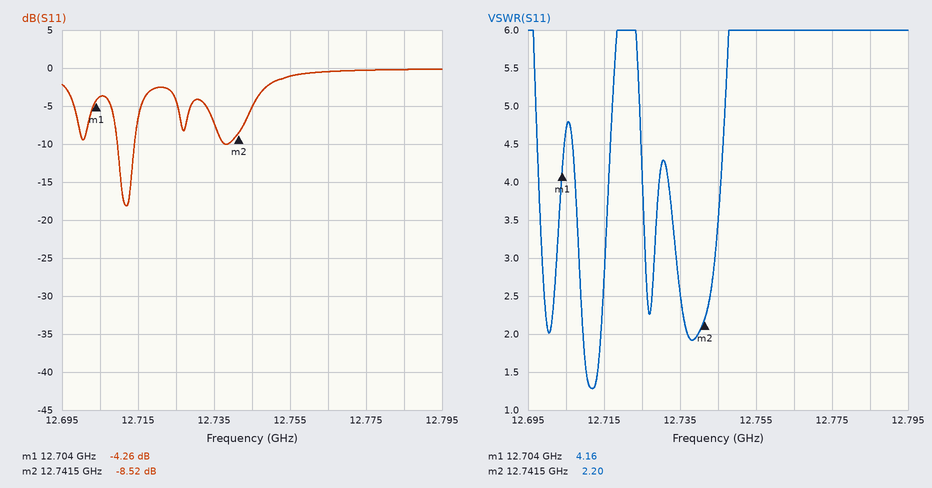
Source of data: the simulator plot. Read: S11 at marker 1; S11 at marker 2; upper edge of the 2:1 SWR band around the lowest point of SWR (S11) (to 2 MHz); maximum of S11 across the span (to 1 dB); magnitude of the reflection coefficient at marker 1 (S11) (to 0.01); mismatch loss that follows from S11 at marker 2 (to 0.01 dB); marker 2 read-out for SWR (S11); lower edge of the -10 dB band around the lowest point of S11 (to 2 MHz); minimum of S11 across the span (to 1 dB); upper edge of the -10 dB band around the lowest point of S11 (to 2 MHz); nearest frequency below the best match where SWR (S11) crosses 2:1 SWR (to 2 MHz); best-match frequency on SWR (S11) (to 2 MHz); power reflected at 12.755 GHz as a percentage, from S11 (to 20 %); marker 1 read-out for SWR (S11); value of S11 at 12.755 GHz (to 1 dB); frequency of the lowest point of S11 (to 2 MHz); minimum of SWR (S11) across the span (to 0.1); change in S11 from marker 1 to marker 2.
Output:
-4.26 dB
-8.52 dB
12.714 GHz
0 dB
0.61
0.66 dB
2.20
12.710 GHz
-18 dB
12.714 GHz
12.710 GHz
12.712 GHz
80 %
4.16
-1 dB
12.712 GHz
1.3
-4.26 dB
